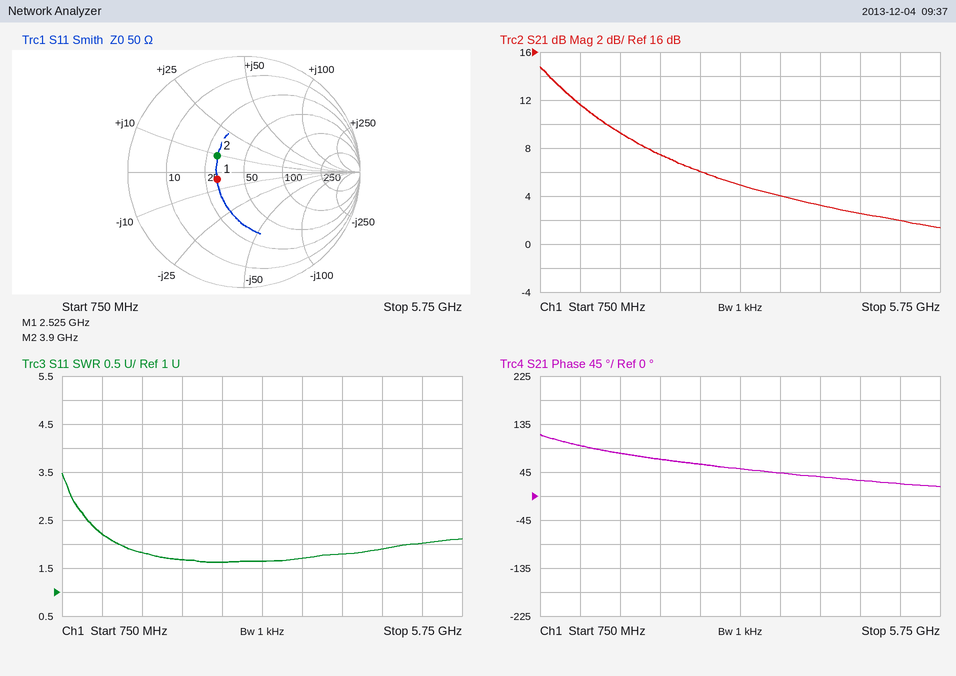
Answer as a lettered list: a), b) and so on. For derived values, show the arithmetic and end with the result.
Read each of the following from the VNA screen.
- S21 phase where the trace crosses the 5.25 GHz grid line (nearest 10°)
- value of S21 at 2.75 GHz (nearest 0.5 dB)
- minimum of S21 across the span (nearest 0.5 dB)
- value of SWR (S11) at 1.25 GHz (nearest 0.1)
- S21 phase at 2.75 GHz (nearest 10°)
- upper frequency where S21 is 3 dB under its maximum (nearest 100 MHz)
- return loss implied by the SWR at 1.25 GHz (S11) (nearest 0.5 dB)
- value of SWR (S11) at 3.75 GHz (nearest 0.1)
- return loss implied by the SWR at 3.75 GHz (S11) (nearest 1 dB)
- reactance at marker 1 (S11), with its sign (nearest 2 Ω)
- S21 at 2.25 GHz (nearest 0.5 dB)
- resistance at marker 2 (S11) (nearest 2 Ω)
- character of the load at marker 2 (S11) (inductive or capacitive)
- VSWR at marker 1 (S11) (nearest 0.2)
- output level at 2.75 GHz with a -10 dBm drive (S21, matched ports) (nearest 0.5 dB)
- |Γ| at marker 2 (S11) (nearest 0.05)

a) 20°
b) 6.0 dB
c) 1.5 dB
d) 2.2
e) 60°
f) 1.2 GHz
g) −20 log10((2.2 − 1)/(2.2 + 1)) ≈ 8.5 dB
h) 1.7
i) −20 log10((1.7 − 1)/(1.7 + 1)) ≈ 12 dB
j) -4 Ω
k) 7.5 dB
l) 30 Ω
m) inductive
n) 1.6
o) -10 dBm + (6.0 dB) = -4.0 dBm
p) 0.25
